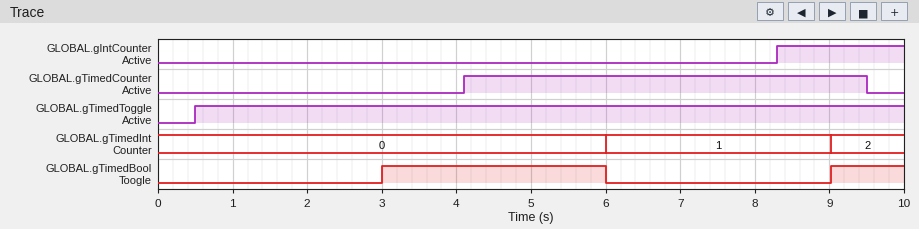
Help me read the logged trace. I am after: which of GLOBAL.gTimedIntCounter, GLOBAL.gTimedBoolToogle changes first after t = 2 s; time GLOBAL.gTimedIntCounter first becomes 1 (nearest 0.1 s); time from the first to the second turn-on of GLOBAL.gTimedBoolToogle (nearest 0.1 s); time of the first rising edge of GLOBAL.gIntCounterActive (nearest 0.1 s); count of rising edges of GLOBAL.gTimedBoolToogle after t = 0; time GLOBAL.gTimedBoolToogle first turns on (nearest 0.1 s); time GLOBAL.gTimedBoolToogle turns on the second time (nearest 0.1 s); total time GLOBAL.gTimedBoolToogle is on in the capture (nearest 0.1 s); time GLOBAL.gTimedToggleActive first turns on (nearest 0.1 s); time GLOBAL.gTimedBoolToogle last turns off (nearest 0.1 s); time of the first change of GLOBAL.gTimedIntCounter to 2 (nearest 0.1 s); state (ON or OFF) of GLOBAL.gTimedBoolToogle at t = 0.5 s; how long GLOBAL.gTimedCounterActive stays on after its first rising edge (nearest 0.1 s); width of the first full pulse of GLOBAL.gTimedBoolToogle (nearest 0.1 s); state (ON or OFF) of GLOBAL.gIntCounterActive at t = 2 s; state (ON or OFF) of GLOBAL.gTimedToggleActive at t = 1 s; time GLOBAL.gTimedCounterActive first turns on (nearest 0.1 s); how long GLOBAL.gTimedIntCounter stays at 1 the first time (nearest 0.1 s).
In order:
GLOBAL.gTimedBoolToogle
6.0 s
6.0 s
8.3 s
2
3.0 s
9.0 s
4.0 s
0.5 s
6.0 s
9.0 s
OFF
5.4 s
3.0 s
OFF
ON
4.1 s
3.0 s
